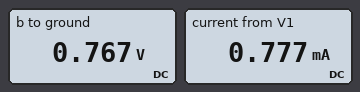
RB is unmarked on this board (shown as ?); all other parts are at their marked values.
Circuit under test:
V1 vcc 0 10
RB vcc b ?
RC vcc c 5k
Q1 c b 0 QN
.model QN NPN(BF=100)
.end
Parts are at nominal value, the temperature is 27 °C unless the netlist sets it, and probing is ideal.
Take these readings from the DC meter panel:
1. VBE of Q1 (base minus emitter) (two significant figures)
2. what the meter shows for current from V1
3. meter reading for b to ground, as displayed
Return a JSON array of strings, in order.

["770 mV", "0.777 mA", "0.767 V"]
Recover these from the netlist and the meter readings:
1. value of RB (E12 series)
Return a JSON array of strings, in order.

["1.2 MΩ"]
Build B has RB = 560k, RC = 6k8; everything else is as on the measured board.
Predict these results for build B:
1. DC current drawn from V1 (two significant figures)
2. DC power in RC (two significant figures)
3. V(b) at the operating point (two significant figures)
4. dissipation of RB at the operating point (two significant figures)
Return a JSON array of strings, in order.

["1.5 mA", "14 mW", "780 mV", "150 µW"]
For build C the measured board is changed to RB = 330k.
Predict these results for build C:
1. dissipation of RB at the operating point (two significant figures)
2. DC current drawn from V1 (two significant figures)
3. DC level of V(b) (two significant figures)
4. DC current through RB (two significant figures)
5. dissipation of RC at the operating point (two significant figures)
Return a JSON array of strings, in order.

["260 µW", "2.0 mA", "790 mV", "28 µA", "19 mW"]
